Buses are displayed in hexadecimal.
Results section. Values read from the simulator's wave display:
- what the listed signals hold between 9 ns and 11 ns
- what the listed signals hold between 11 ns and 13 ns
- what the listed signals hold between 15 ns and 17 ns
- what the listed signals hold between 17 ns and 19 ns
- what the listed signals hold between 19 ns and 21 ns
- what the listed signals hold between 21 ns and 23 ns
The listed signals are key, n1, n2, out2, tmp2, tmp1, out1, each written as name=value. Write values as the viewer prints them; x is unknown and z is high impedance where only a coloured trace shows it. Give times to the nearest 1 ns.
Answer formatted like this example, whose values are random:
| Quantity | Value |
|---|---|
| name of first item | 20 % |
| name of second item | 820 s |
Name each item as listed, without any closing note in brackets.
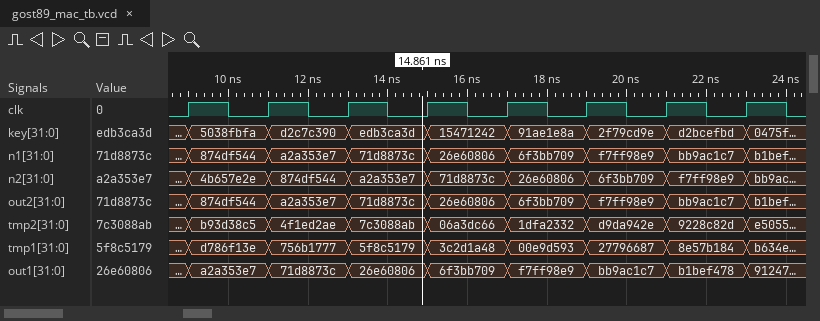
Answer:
| Quantity | Value |
|---|---|
| what the listed signals hold between 9 ns and 11 ns | key=5038fbfa, n1=874df544, n2=4b657e2e, out2=874df544, tmp2=b93d38c5, tmp1=d786f13e, out1=a2a353e7 |
| what the listed signals hold between 11 ns and 13 ns | key=d2c7c390, n1=a2a353e7, n2=874df544, out2=a2a353e7, tmp2=4f1ed2ae, tmp1=756b1777, out1=71d8873c |
| what the listed signals hold between 15 ns and 17 ns | key=15471242, n1=26e60806, n2=71d8873c, out2=26e60806, tmp2=06a3dc66, tmp1=3c2d1a48, out1=6f3bb709 |
| what the listed signals hold between 17 ns and 19 ns | key=91ae1e8a, n1=6f3bb709, n2=26e60806, out2=6f3bb709, tmp2=1dfa2332, tmp1=00e9d593, out1=f7ff98e9 |
| what the listed signals hold between 19 ns and 21 ns | key=2f79cd9e, n1=f7ff98e9, n2=6f3bb709, out2=f7ff98e9, tmp2=d9da942e, tmp1=27796687, out1=bb9ac1c7 |
| what the listed signals hold between 21 ns and 23 ns | key=d2bcefbd, n1=bb9ac1c7, n2=f7ff98e9, out2=bb9ac1c7, tmp2=9228c82d, tmp1=8e57b184, out1=b1bef478 |
